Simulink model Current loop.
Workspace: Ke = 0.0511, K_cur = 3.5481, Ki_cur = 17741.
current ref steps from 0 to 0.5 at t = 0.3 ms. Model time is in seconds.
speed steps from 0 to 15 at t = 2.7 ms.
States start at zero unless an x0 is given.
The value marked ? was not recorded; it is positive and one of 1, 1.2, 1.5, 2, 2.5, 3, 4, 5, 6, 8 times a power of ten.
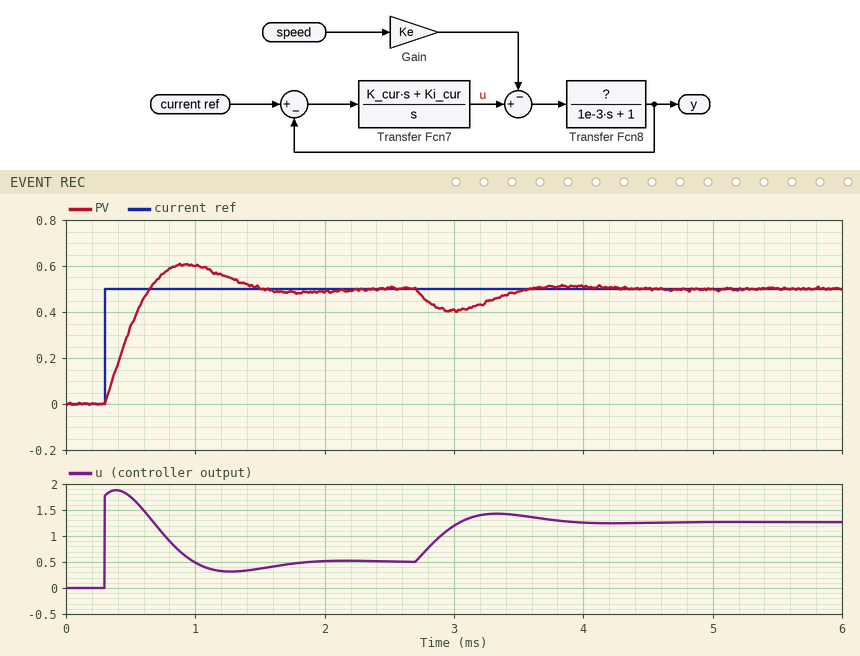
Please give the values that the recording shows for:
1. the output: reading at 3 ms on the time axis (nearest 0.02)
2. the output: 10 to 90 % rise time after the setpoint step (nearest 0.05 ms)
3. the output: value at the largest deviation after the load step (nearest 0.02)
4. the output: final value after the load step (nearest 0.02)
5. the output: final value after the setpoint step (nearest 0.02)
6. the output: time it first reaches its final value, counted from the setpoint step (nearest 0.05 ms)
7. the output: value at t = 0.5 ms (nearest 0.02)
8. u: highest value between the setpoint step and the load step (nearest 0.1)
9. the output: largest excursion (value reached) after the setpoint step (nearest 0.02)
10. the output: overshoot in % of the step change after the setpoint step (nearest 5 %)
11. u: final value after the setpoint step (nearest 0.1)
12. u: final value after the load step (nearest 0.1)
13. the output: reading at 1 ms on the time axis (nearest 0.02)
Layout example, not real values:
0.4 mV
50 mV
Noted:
0.40
0.25 ms
0.40
0.50
0.50
0.35 ms
0.34
1.9
0.60
20 %
0.5
1.3
0.60
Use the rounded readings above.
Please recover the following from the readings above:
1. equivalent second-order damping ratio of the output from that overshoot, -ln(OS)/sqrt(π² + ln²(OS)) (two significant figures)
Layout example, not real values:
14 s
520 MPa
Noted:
0.46
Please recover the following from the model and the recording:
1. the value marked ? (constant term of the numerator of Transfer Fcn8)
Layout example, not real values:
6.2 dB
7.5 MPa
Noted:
1
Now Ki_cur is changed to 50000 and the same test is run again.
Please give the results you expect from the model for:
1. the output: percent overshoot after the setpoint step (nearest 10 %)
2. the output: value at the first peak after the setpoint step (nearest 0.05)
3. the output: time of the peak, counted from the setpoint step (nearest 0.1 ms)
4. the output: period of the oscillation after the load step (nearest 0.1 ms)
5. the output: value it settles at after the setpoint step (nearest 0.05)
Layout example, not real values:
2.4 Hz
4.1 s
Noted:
40 %
0.70
0.4 ms
0.9 ms
0.50
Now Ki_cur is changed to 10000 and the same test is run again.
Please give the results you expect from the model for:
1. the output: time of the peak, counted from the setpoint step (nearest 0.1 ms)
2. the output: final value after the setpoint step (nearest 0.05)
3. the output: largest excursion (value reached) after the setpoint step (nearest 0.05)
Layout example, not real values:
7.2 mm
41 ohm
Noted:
0.8 ms
0.50
0.55
